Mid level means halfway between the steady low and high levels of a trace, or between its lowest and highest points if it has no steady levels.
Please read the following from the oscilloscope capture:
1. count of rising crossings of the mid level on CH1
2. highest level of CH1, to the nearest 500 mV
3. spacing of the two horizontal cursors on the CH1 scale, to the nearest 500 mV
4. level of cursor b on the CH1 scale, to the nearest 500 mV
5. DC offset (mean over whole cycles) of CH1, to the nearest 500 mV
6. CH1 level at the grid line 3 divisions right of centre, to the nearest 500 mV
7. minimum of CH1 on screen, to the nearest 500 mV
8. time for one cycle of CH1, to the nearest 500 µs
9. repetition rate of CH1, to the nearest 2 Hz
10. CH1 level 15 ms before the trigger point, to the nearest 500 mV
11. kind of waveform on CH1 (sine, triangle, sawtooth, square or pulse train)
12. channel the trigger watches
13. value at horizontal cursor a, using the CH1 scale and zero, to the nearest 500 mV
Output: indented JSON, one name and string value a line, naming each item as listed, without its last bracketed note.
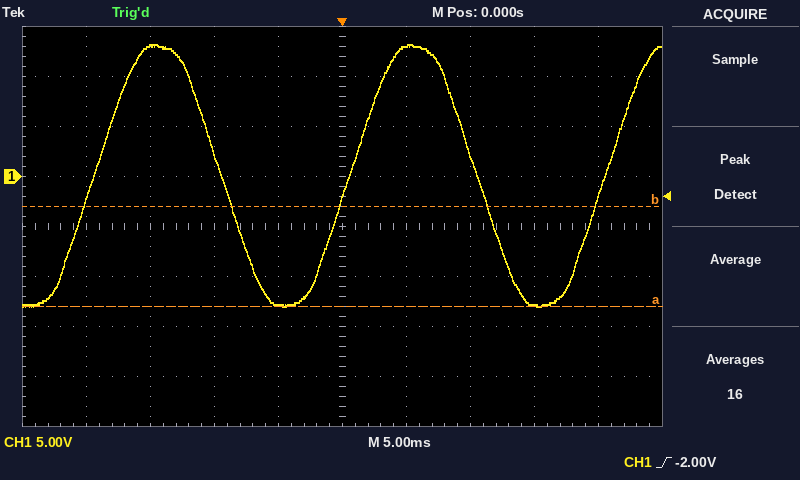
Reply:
{
  "count of rising crossings of the mid level on CH1": "3",
  "highest level of CH1, to the nearest 500 mV": "13.0 V",
  "spacing of the two horizontal cursors on the CH1 scale, to the nearest 500 mV": "10.0 V",
  "level of cursor b on the CH1 scale, to the nearest 500 mV": "-3.0 V",
  "DC offset (mean over whole cycles) of CH1, to the nearest 500 mV": "0.0 V",
  "CH1 level at the grid line 3 divisions right of centre, to the nearest 500 mV": "-13.0 V",
  "minimum of CH1 on screen, to the nearest 500 mV": "-13.0 V",
  "time for one cycle of CH1, to the nearest 500 µs": "20.0 ms",
  "repetition rate of CH1, to the nearest 2 Hz": "50 Hz",
  "CH1 level 15 ms before the trigger point, to the nearest 500 mV": "13.0 V",
  "kind of waveform on CH1": "sine",
  "channel the trigger watches": "CH1",
  "value at horizontal cursor a, using the CH1 scale and zero, to the nearest 500 mV": "-13.0 V"
}
